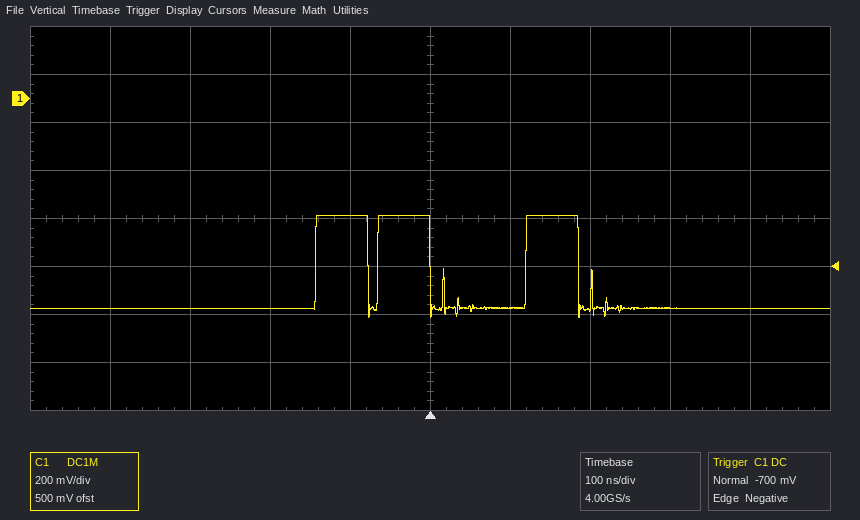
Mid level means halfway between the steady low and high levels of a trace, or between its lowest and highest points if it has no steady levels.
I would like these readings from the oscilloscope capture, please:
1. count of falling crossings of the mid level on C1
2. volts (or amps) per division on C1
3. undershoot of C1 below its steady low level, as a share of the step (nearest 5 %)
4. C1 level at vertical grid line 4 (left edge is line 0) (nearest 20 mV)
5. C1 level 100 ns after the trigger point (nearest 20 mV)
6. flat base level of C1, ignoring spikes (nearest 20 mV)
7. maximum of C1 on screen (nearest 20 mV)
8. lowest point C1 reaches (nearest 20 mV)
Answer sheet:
3
200 mV
10 %
-480 mV
-880 mV
-880 mV
-480 mV
-920 mV
